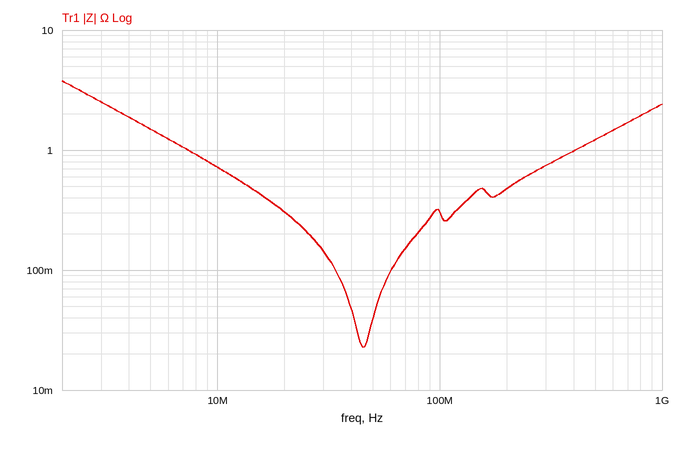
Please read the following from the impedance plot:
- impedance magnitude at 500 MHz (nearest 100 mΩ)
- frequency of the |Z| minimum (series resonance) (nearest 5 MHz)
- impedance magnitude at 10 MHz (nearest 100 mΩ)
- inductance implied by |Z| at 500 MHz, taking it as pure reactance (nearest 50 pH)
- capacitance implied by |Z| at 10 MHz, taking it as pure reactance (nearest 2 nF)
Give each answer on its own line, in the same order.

1.2 Ω
45 MHz
700 mΩ
400 pH
22 nF
